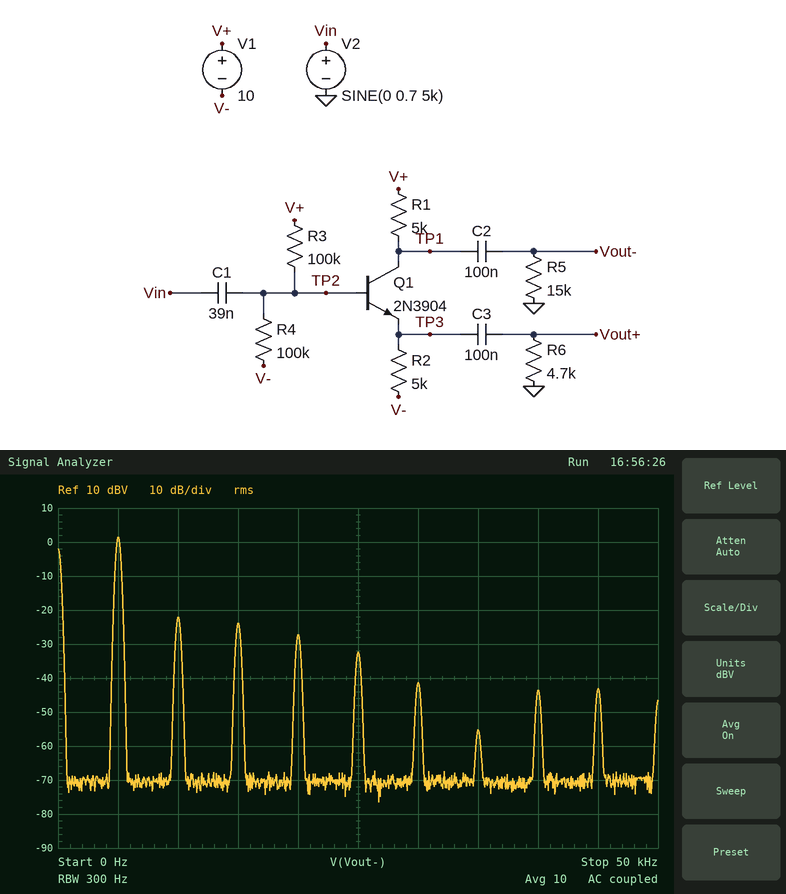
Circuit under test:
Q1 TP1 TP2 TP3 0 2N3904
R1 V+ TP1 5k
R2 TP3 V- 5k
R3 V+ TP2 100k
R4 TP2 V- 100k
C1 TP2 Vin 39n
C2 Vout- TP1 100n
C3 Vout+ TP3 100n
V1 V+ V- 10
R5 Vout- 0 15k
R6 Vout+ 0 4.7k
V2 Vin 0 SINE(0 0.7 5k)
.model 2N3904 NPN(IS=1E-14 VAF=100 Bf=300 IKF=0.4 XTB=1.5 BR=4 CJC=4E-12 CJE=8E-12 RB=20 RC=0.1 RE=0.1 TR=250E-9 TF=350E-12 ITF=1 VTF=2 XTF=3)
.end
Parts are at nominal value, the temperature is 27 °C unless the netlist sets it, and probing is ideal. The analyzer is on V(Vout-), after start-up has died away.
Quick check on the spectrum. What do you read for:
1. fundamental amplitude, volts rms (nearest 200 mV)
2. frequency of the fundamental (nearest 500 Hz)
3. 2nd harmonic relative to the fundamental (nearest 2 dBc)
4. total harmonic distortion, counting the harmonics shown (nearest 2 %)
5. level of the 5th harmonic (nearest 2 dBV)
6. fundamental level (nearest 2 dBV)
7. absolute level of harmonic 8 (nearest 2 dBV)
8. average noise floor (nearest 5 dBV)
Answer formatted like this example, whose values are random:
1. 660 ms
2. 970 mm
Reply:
1. 1.2 V
2. 5.0 kHz
3. -24 dBc
4. 10 %
5. -32 dBV
6. 2 dBV
7. -44 dBV
8. -70 dBV
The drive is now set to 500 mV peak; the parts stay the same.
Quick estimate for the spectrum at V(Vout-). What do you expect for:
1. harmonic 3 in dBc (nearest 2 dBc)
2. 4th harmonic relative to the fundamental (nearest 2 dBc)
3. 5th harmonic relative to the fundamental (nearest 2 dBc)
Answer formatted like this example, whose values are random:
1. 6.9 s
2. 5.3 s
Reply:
1. -34 dBc
2. -36 dBc
3. -38 dBc
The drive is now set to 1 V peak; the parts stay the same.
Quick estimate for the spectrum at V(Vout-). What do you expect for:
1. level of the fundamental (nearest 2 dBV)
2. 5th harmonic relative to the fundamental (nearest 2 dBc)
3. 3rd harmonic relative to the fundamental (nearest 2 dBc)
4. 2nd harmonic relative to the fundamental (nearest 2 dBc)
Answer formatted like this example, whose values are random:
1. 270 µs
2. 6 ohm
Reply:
1. 4 dBV
2. -36 dBc
3. -22 dBc
4. -20 dBc
